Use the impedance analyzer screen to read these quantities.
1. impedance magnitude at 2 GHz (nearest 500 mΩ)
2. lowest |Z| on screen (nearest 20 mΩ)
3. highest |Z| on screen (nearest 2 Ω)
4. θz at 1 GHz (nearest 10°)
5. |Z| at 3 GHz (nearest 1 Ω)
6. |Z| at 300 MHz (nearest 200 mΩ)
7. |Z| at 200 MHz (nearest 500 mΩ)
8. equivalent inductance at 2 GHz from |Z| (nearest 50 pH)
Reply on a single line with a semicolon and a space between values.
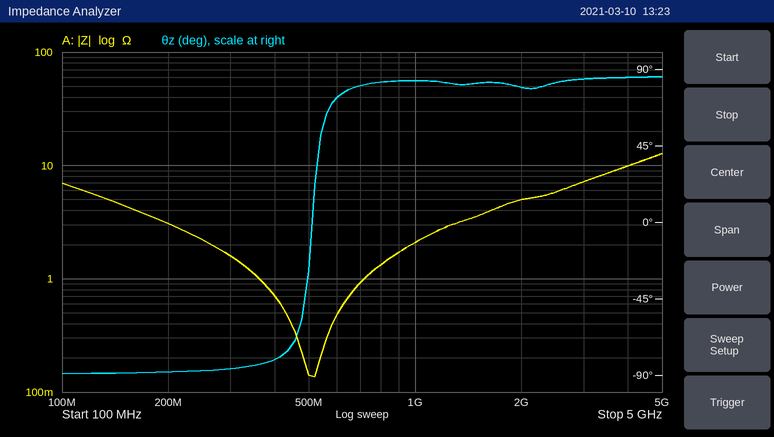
5.0 Ω; 140 mΩ; 12 Ω; 80°; 7 Ω; 1.6 Ω; 3.0 Ω; 400 pH
